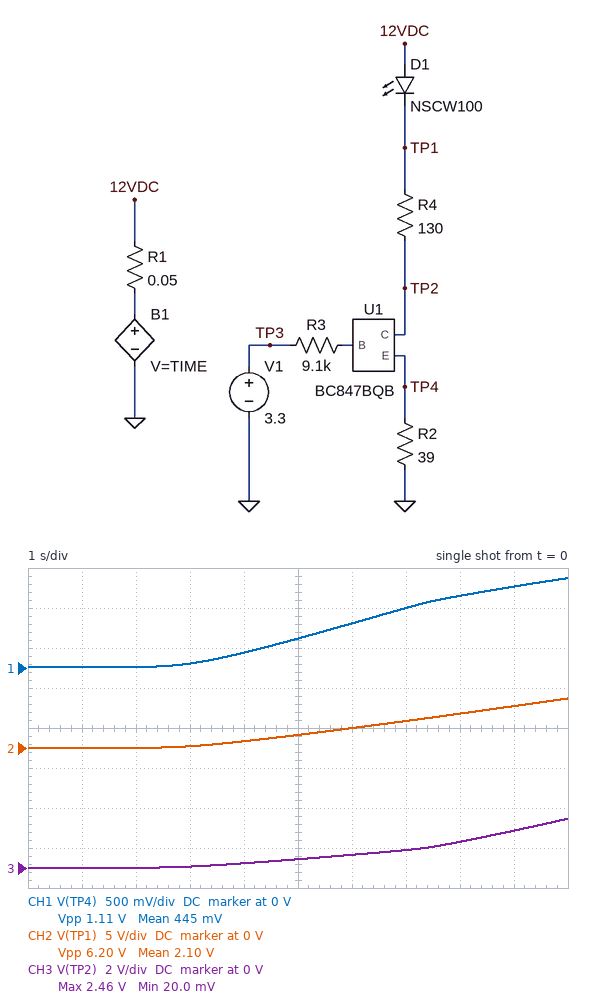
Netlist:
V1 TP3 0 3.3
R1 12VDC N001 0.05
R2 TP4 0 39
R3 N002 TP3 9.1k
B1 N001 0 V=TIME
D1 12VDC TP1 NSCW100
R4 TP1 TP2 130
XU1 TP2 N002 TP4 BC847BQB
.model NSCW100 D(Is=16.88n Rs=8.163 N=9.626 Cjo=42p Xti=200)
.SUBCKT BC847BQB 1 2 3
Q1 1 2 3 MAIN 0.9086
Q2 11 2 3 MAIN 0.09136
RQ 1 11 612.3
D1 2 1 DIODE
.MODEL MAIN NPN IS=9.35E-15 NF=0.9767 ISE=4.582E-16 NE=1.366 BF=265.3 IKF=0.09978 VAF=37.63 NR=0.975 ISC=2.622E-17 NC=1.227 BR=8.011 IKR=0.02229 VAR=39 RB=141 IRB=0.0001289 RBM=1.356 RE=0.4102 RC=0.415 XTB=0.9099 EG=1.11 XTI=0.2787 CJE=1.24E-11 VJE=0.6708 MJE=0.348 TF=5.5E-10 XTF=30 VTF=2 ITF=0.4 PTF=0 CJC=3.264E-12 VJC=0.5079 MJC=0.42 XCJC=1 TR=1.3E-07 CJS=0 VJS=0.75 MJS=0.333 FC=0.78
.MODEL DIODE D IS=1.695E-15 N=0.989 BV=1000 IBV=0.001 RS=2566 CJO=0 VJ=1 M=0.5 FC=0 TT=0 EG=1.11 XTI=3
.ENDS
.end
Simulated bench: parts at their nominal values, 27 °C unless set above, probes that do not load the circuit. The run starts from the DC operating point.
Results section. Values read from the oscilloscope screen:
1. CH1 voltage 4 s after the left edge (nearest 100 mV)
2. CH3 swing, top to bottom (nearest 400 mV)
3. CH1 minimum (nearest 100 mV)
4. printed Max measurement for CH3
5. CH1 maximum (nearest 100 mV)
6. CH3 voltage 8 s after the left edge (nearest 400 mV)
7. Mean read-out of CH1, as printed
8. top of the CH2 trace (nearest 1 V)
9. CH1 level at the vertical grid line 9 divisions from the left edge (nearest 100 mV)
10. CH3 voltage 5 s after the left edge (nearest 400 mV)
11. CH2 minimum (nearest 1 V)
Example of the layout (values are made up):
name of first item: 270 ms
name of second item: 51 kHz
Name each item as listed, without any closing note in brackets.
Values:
CH1 voltage 4 s after the left edge: 200 mV
CH3 swing, top to bottom: 2.4 V
CH1 minimum: 0 V
printed Max measurement for CH3: 2.46 V
CH1 maximum: 1.1 V
CH3 voltage 8 s after the left edge: 1.2 V
Mean read-out of CH1, as printed: 445 mV
top of the CH2 trace: 6 V
CH1 level at the vertical grid line 9 divisions from the left edge: 1.0 V
CH3 voltage 5 s after the left edge: 400 mV
CH2 minimum: 0 V
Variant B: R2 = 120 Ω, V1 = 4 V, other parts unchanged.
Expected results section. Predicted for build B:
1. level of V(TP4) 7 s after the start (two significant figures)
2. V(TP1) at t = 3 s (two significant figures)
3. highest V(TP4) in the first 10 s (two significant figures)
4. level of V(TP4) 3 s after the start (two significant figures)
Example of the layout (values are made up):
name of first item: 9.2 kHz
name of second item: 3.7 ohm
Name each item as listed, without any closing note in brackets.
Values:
level of V(TP4) 7 s after the start: 1.6 V
V(TP1) at t = 3 s: 280 mV
highest V(TP4) in the first 10 s: 2.4 V
level of V(TP4) 3 s after the start: 150 mV
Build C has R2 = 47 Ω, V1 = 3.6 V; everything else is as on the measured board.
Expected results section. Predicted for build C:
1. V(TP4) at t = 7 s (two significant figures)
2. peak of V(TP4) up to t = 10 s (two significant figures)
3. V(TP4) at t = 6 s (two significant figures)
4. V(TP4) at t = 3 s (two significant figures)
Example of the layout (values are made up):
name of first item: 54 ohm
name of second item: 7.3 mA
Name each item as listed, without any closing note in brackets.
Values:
V(TP4) at t = 7 s: 870 mV
peak of V(TP4) up to t = 10 s: 1.3 V
V(TP4) at t = 6 s: 650 mV
V(TP4) at t = 3 s: 67 mV
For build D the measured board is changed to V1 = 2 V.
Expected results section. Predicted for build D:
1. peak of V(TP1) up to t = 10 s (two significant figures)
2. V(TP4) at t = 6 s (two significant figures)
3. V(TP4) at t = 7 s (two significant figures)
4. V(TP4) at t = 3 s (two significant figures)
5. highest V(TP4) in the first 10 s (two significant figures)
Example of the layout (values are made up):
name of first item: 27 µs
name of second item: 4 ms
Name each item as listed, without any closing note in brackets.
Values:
peak of V(TP1) up to t = 10 s: 6.4 V
V(TP4) at t = 6 s: 500 mV
V(TP4) at t = 7 s: 610 mV
V(TP4) at t = 3 s: 50 mV
highest V(TP4) in the first 10 s: 650 mV
